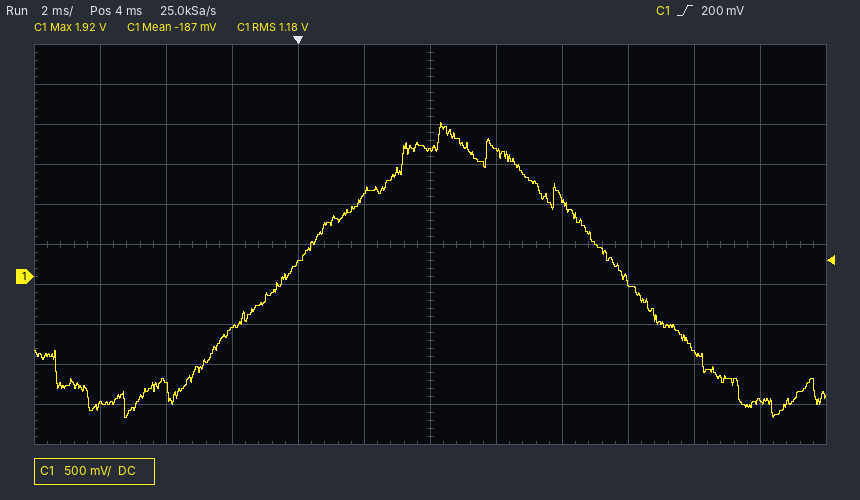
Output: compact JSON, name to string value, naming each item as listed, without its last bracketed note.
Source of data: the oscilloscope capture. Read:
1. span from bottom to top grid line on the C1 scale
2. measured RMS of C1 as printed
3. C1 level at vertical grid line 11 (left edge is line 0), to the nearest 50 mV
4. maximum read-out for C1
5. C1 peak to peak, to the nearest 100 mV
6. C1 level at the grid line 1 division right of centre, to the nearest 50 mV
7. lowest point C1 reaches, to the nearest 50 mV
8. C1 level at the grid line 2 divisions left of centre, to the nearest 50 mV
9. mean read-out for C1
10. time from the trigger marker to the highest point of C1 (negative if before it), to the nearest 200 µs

{"span from bottom to top grid line on the C1 scale": "5 V", "measured RMS of C1 as printed": "1.18 V", "C1 level at vertical grid line 11 (left edge is line 0), to the nearest 50 mV": "-1.55 V", "maximum read-out for C1": "1.92 V", "C1 peak to peak, to the nearest 100 mV": "3.70 V", "C1 level at the grid line 1 division right of centre, to the nearest 50 mV": "1.60 V", "lowest point C1 reaches, to the nearest 50 mV": "-1.75 V", "C1 level at the grid line 2 divisions left of centre, to the nearest 50 mV": "150 mV", "mean read-out for C1": "-187 mV", "time from the trigger marker to the highest point of C1 (negative if before it), to the nearest 200 µs": "+4.4 ms"}
